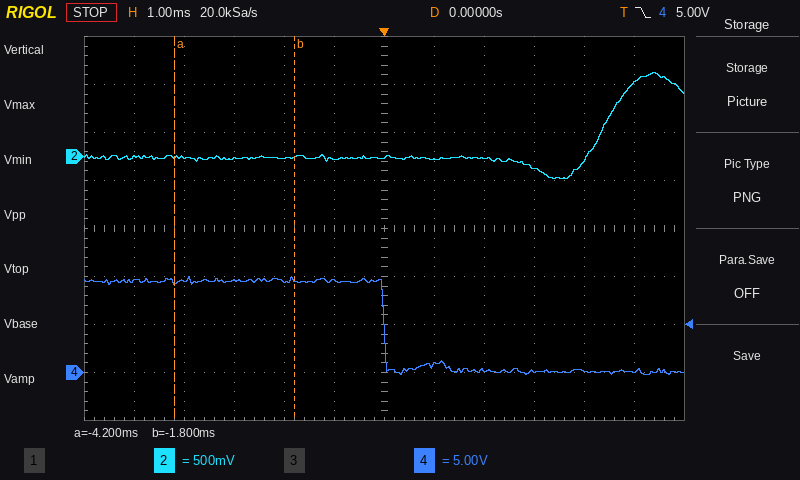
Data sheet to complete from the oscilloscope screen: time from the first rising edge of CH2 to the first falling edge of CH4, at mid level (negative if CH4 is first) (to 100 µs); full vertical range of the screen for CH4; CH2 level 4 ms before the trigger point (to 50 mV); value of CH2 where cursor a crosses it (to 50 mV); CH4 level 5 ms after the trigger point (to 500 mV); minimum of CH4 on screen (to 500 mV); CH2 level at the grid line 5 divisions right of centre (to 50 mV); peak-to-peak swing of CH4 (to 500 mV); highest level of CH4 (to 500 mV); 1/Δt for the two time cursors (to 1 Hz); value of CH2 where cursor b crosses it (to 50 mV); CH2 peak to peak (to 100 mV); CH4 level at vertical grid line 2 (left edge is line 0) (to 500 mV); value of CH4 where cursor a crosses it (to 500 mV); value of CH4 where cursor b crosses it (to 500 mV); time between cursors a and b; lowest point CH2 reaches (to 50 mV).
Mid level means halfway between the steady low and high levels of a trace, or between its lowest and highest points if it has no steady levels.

-4.4 ms
40 V
0 mV
0 mV
0.0 V
0.0 V
750 mV
10.0 V
10.0 V
417 Hz
0 mV
1.10 V
9.5 V
9.5 V
9.5 V
2.4 ms
-250 mV
